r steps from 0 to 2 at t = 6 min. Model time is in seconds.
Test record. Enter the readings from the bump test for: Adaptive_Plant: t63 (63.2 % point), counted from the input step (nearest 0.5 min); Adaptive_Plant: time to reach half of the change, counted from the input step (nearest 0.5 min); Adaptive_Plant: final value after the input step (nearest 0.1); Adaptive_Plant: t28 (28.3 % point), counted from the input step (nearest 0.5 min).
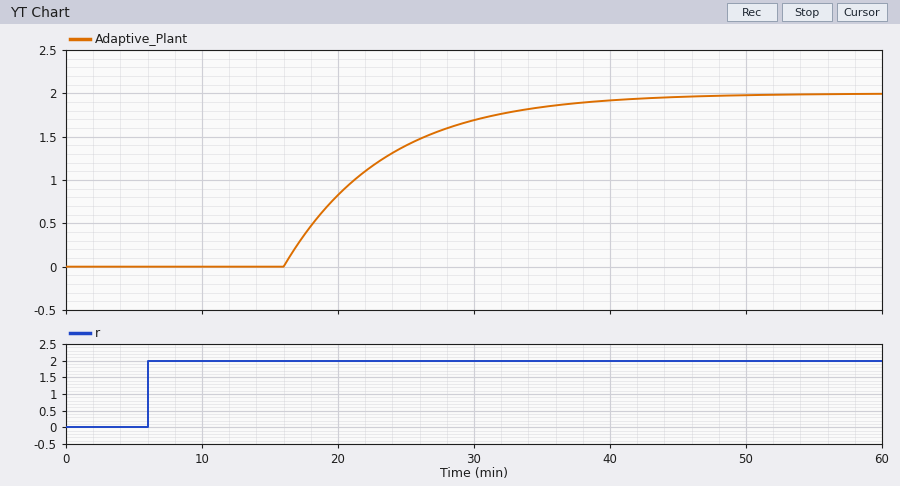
17.5 min
15.0 min
2.0
12.5 min
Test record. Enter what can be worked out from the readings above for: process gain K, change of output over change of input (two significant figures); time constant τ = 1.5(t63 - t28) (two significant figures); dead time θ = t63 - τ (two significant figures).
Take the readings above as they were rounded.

1.0
7.5 min
10 min
